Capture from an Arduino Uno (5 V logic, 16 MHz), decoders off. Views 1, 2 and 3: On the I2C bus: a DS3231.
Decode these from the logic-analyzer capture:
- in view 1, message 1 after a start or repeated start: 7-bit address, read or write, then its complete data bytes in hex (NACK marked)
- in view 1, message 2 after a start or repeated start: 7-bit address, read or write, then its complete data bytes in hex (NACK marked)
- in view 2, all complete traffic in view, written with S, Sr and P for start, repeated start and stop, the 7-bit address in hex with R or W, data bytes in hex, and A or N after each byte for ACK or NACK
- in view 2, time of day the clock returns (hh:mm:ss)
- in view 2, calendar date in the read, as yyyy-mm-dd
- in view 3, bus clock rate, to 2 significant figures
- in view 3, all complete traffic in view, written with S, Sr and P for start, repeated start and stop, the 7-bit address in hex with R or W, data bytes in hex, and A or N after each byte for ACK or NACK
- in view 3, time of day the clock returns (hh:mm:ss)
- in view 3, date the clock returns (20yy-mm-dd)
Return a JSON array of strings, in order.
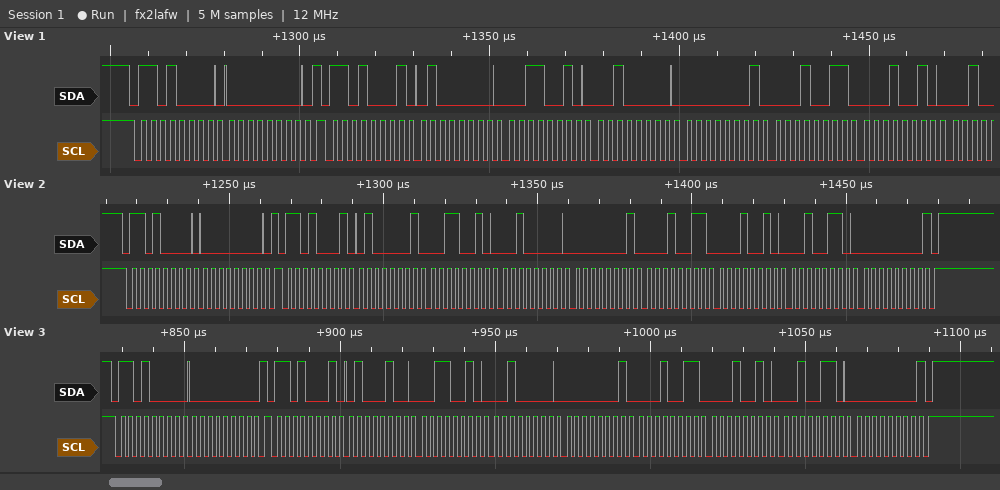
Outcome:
["0x68 write: 00", "0x68 read: 40 32 20 01 13 12", "S 68W A 00 A Sr 68R A 41 A 32 A 20 A 01 A 13 A 12 A 26 A 00 N P", "20:32:41", "2026-12-13", "400 kHz", "S 68W A 00 A Sr 68R A 44 A 32 A 20 A 01 A 13 A 12 A 26 A 00 N P", "20:32:44", "2026-12-13"]
